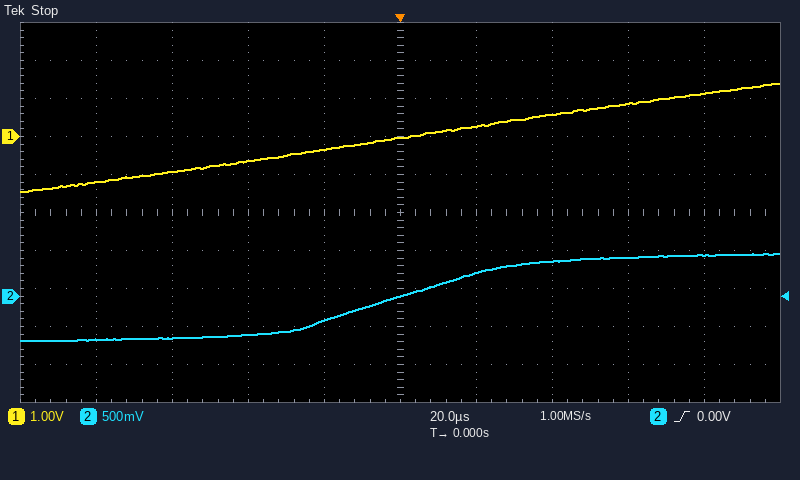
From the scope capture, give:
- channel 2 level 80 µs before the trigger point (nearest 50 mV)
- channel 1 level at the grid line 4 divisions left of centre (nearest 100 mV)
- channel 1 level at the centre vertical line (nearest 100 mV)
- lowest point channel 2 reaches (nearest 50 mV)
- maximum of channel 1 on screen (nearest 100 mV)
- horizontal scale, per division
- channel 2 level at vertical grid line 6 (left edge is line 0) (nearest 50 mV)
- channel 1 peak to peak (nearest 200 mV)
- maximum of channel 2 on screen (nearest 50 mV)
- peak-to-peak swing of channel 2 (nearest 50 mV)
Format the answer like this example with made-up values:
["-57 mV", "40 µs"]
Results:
["-550 mV", "-1.2 V", "0.0 V", "-600 mV", "1.4 V", "20 µs", "300 mV", "2.8 V", "550 mV", "1.15 V"]
